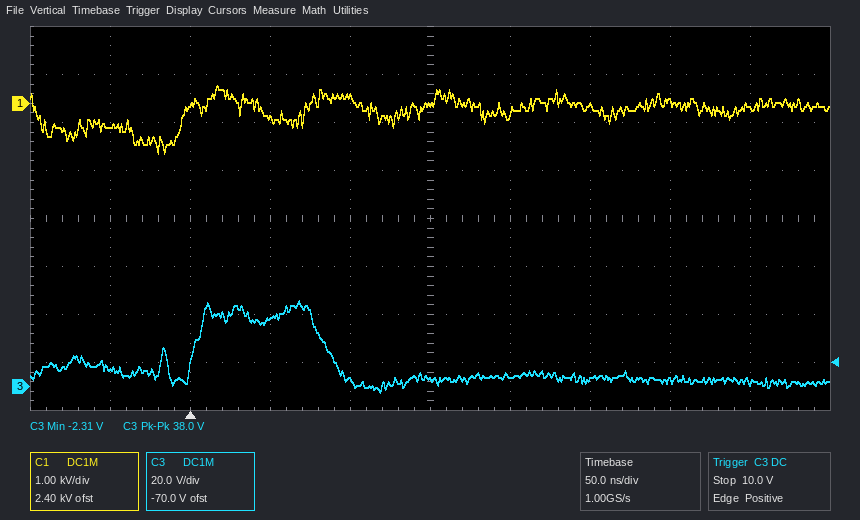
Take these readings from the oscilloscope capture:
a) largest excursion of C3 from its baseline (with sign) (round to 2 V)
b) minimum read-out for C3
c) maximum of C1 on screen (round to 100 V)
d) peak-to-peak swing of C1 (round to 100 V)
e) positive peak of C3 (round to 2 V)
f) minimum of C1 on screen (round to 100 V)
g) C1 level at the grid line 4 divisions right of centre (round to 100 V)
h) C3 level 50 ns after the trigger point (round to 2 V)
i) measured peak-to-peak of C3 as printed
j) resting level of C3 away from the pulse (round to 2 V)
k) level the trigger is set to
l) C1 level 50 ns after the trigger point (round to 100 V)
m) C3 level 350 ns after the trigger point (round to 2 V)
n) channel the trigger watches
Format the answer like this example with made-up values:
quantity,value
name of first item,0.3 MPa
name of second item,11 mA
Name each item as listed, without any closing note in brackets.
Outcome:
quantity,value
largest excursion of C3 from its baseline (with sign),+32 V
minimum read-out for C3,-2.31 V
maximum of C1 on screen,400 V
peak-to-peak swing of C1,1.4 kV
positive peak of C3,36 V
minimum of C1 on screen,-1.0 kV
C1 level at the grid line 4 divisions right of centre,-100 V
C3 level 50 ns after the trigger point,28 V
measured peak-to-peak of C3 as printed,38.0 V
resting level of C3 away from the pulse,4 V
level the trigger is set to,10.0 V
C1 level 50 ns after the trigger point,-300 V
C3 level 350 ns after the trigger point,2 V
channel the trigger watches,C3
